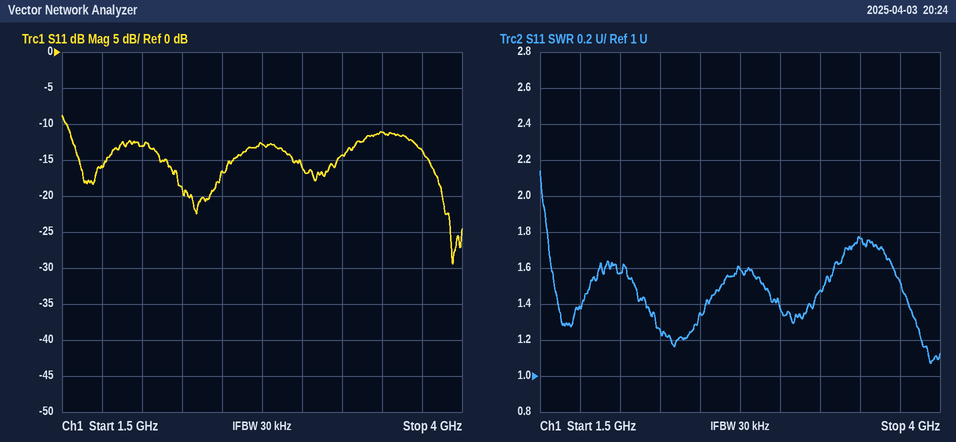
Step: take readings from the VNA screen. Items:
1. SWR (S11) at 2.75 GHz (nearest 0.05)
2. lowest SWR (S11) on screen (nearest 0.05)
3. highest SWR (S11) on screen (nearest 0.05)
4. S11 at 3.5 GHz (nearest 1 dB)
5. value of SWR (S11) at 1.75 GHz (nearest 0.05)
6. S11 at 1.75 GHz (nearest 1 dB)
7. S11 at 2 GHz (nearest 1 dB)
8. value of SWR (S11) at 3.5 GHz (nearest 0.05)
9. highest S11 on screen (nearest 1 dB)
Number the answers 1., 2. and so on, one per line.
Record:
1. 1.60
2. 1.05
3. 2.15
4. -11 dB
5. 1.40
6. -16 dB
7. -13 dB
8. 1.75
9. -9 dB
